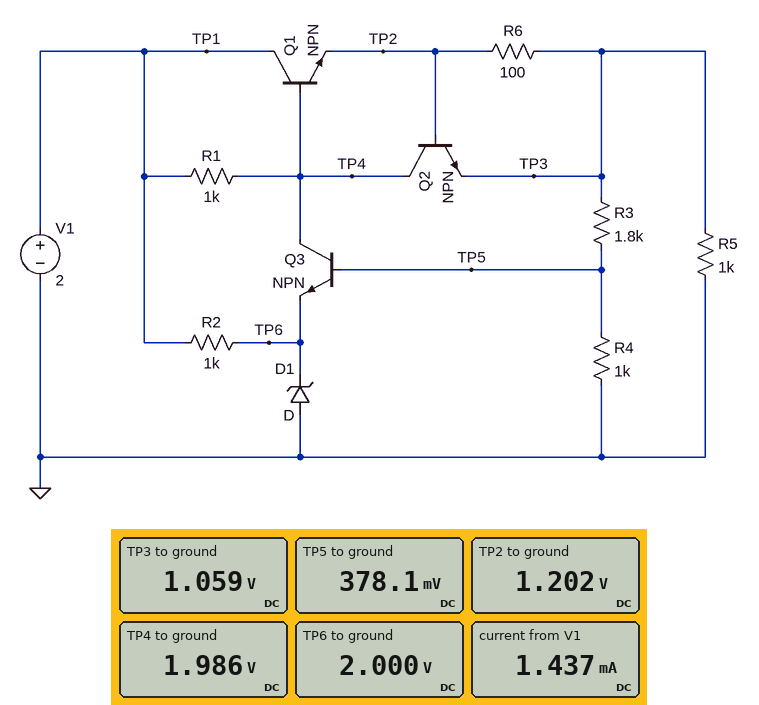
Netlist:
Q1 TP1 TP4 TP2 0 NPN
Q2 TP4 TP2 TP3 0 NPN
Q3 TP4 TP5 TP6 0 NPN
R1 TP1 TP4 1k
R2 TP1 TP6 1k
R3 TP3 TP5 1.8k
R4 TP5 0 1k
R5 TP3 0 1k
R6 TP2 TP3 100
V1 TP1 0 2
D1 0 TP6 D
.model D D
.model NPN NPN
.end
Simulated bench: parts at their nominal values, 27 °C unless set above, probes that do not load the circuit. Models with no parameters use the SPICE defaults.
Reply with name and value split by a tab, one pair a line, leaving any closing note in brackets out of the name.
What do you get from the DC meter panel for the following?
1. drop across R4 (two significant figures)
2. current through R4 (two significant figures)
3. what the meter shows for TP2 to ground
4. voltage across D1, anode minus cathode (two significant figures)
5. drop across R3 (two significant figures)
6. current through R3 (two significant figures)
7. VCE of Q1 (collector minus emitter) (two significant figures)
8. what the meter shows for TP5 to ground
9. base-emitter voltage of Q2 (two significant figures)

drop across R4	380 mV
current through R4	380 µA
what the meter shows for TP2 to ground	1.202 V
voltage across D1, anode minus cathode	-2.0 V
drop across R3	680 mV
current through R3	380 µA
VCE of Q1 (collector minus emitter)	800 mV
what the meter shows for TP5 to ground	378.1 mV
base-emitter voltage of Q2	140 mV
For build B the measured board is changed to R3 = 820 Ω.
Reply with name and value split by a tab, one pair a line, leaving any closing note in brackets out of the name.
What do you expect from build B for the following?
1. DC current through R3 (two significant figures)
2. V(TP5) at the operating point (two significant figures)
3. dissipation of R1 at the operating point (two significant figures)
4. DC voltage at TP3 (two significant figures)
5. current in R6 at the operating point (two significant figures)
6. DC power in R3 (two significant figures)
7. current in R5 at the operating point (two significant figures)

DC current through R3	570 µA
V(TP5) at the operating point	570 mV
dissipation of R1 at the operating point	250 nW
DC voltage at TP3	1.0 V
current in R6 at the operating point	1.6 mA
DC power in R3	270 µW
current in R5 at the operating point	1.0 mA
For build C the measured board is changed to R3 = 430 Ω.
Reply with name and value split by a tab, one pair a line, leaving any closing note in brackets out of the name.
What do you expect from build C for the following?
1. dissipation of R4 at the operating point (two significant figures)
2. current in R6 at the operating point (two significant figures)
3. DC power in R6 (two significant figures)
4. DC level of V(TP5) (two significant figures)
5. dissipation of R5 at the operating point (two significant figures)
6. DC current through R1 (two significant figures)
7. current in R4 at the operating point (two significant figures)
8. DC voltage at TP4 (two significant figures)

dissipation of R4 at the operating point	510 µW
current in R6 at the operating point	1.7 mA
DC power in R6	300 µW
DC level of V(TP5)	710 mV
dissipation of R5 at the operating point	1.0 mW
DC current through R1	17 µA
current in R4 at the operating point	710 µA
DC voltage at TP4	2.0 V
